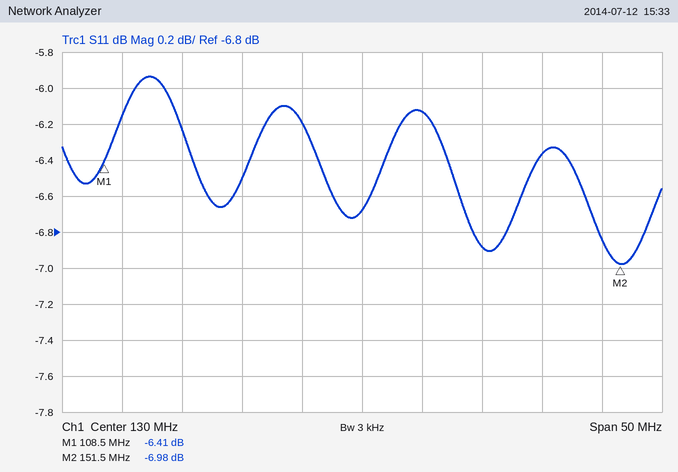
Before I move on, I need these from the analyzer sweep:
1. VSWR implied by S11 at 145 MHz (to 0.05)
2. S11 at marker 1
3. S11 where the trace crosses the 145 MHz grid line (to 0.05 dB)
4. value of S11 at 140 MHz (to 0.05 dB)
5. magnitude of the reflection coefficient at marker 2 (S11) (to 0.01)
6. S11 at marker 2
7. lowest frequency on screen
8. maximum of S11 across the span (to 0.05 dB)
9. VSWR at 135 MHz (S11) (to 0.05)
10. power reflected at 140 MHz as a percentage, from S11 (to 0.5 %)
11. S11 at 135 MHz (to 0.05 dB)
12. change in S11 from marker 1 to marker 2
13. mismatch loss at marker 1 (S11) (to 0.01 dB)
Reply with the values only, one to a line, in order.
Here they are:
2.85
-6.41 dB
-6.35 dB
-6.90 dB
0.45
-6.98 dB
105 MHz
-5.95 dB
2.95
20.5 %
-6.15 dB
-0.57 dB
1.13 dB
